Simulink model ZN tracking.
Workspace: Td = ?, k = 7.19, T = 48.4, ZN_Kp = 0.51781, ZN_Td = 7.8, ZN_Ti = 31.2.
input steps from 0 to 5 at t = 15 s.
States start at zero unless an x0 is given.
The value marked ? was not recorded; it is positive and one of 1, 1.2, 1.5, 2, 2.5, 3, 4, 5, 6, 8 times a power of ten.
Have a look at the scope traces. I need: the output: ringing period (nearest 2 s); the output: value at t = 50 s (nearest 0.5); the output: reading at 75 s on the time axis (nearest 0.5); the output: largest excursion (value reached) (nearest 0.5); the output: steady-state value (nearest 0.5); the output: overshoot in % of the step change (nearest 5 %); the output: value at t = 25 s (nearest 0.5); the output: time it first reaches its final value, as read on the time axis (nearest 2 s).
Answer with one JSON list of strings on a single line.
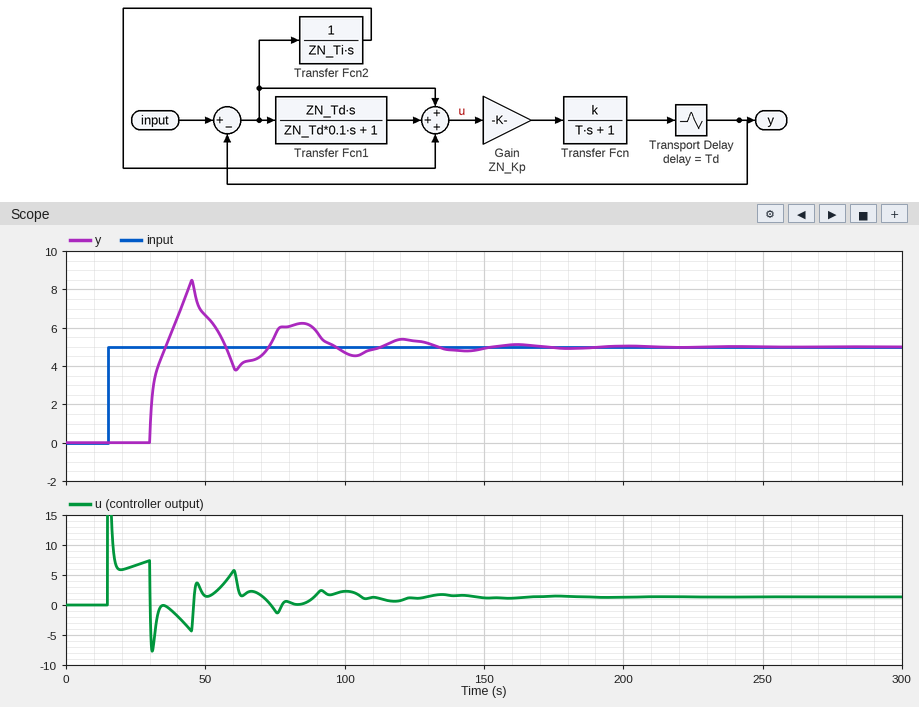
["40 s", "6.5", "5.5", "8.5", "5.0", "70 %", "0.0", "36 s"]
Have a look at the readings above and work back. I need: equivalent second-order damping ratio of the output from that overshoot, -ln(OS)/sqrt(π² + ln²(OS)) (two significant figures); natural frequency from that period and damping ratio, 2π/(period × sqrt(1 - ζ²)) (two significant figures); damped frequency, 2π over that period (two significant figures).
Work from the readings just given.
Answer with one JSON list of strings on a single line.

["0.11", "0.16 rad/s", "0.16 rad/s"]
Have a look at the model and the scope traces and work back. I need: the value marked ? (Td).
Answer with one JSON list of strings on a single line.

["15"]
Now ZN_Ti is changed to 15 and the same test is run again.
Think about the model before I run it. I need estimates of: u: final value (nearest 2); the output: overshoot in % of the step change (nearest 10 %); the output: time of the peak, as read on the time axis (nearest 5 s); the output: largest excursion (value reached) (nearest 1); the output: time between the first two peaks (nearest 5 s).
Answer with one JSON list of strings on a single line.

["2", "100 %", "45 s", "10", "95 s"]
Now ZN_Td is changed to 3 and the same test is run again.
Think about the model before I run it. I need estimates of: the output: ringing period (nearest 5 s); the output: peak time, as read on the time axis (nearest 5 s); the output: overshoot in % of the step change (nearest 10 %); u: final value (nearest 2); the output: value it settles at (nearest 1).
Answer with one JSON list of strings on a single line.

["65 s", "55 s", "60 %", "2", "5"]
